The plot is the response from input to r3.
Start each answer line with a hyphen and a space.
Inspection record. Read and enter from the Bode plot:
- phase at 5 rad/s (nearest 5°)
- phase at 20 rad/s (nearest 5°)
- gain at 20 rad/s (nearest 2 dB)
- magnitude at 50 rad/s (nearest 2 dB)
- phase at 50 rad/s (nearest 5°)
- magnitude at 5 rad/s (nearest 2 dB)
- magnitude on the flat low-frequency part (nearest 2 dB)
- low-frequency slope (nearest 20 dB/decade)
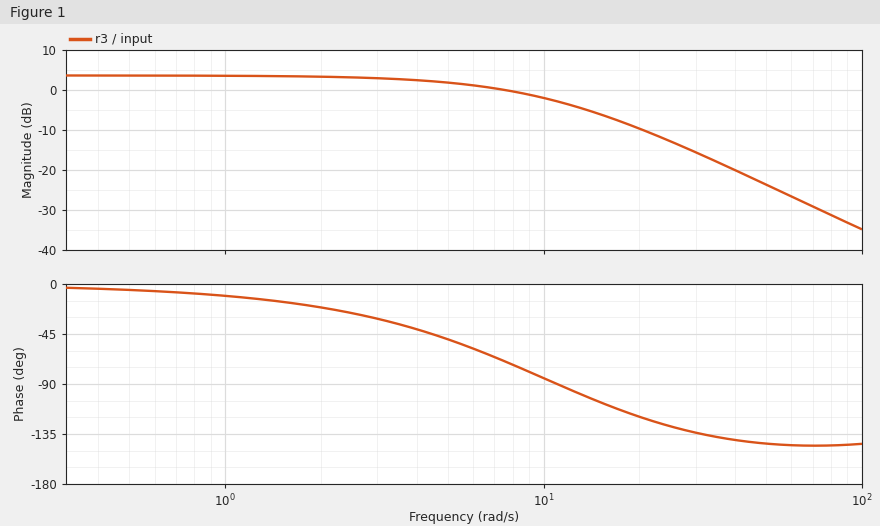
- -50°
- -120°
- -10 dB
- -24 dB
- -145°
- 2 dB
- 4 dB
- 0 dB/decade
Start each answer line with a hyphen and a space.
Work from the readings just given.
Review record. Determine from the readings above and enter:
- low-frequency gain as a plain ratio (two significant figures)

- 1.6
